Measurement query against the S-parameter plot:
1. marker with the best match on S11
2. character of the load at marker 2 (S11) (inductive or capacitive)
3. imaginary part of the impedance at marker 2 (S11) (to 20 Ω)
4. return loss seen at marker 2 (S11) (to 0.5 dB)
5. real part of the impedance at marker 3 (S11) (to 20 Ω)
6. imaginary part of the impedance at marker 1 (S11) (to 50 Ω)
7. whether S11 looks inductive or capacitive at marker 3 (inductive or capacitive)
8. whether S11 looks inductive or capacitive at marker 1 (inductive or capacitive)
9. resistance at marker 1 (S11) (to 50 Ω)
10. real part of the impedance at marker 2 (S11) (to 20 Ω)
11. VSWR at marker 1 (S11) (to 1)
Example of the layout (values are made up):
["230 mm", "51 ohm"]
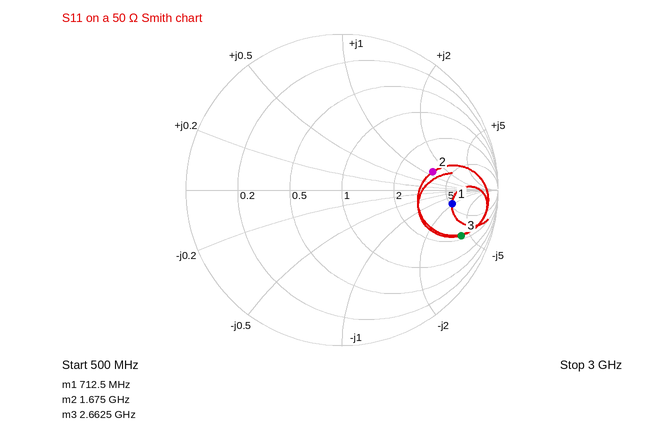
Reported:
["marker 2", "inductive", "+60 Ω", "4.5 dB", "120 Ω", "-100 Ω", "capacitive", "capacitive", "250 Ω", "180 Ω", "6"]
